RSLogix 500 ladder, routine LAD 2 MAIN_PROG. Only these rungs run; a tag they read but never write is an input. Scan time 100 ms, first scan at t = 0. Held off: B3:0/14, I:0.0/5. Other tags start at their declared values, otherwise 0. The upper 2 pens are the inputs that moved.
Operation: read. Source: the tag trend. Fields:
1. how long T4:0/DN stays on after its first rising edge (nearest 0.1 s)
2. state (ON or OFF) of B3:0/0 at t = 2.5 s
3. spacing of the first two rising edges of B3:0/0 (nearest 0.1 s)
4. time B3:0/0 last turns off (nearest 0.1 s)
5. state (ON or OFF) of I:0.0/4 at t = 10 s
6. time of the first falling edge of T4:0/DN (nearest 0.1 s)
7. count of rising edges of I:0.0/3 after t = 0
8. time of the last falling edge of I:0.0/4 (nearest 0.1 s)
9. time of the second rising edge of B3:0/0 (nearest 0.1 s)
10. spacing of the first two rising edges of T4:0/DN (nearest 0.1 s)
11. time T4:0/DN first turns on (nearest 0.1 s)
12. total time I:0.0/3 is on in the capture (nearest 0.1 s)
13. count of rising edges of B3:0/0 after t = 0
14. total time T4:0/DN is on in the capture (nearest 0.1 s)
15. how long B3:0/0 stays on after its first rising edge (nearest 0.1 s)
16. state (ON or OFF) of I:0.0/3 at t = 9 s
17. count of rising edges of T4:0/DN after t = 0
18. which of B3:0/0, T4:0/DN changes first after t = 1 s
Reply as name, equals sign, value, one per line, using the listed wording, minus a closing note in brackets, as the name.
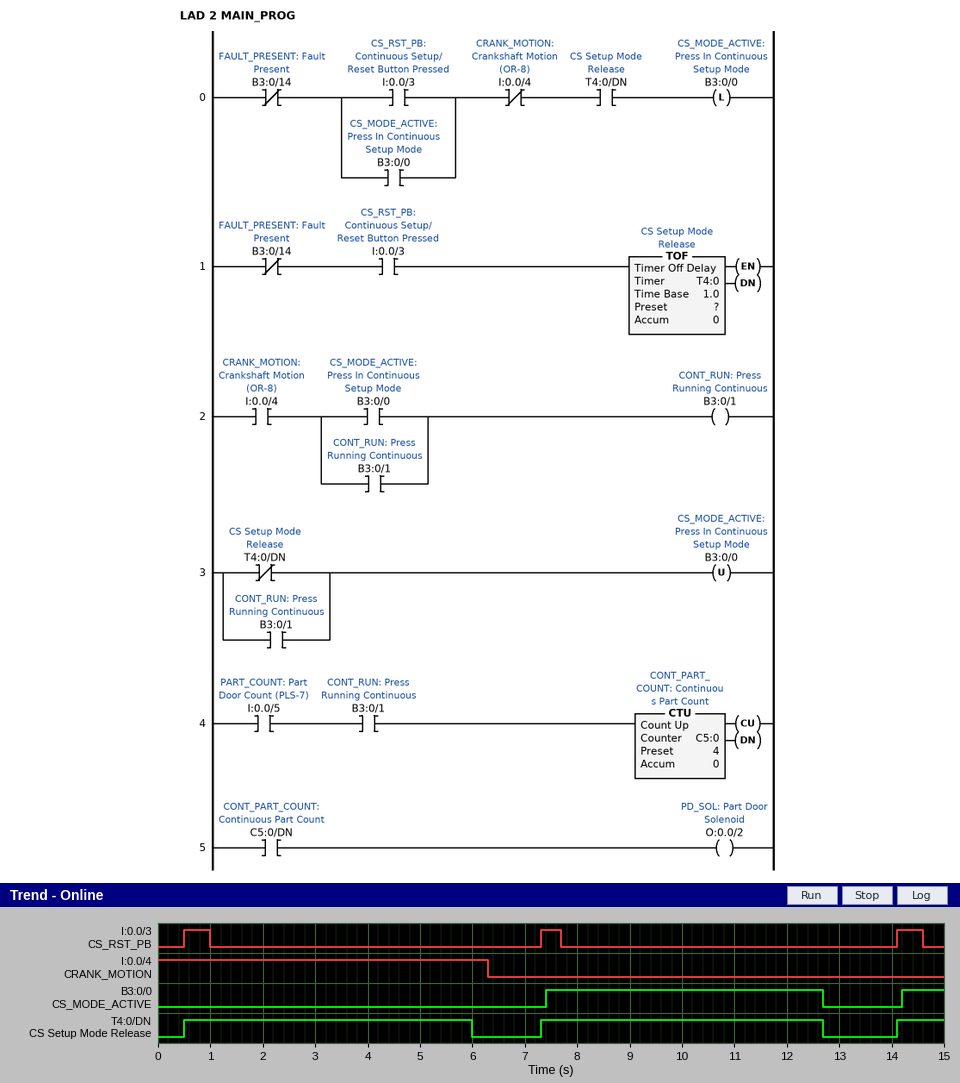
how long T4:0/DN stays on after its first rising edge = 5.5 s
state (ON or OFF) of B3:0/0 at t = 2.5 s = OFF
spacing of the first two rising edges of B3:0/0 = 6.8 s
time B3:0/0 last turns off = 12.7 s
state (ON or OFF) of I:0.0/4 at t = 10 s = OFF
time of the first falling edge of T4:0/DN = 6.0 s
count of rising edges of I:0.0/3 after t = 0 = 3
time of the last falling edge of I:0.0/4 = 6.3 s
time of the second rising edge of B3:0/0 = 14.2 s
spacing of the first two rising edges of T4:0/DN = 6.8 s
time T4:0/DN first turns on = 0.5 s
total time I:0.0/3 is on in the capture = 1.4 s
count of rising edges of B3:0/0 after t = 0 = 2
total time T4:0/DN is on in the capture = 11.8 s
how long B3:0/0 stays on after its first rising edge = 5.3 s
state (ON or OFF) of I:0.0/3 at t = 9 s = OFF
count of rising edges of T4:0/DN after t = 0 = 3
which of B3:0/0, T4:0/DN changes first after t = 1 s = T4:0/DN
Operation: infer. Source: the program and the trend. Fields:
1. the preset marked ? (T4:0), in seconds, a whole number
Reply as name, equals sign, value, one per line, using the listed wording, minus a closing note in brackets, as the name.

the preset marked ? (T4:0), in seconds, a whole number = 5 s
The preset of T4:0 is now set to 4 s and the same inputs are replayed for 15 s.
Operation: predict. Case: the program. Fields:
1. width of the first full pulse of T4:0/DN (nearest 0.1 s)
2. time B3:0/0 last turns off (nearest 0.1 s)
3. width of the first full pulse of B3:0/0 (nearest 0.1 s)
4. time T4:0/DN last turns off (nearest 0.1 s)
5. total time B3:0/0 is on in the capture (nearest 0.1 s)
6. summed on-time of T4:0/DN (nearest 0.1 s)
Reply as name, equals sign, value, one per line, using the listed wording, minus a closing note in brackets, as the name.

width of the first full pulse of T4:0/DN = 4.5 s
time B3:0/0 last turns off = 11.7 s
width of the first full pulse of B3:0/0 = 4.3 s
time T4:0/DN last turns off = 11.7 s
total time B3:0/0 is on in the capture = 5.1 s
summed on-time of T4:0/DN = 9.8 s
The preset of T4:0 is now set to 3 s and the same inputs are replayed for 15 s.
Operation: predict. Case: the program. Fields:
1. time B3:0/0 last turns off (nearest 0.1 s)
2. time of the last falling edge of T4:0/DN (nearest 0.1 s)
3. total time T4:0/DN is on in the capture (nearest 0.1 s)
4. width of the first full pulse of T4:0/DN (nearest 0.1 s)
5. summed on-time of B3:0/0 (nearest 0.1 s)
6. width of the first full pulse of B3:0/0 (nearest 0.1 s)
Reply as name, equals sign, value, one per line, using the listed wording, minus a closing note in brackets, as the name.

time B3:0/0 last turns off = 10.7 s
time of the last falling edge of T4:0/DN = 10.7 s
total time T4:0/DN is on in the capture = 7.8 s
width of the first full pulse of T4:0/DN = 3.5 s
summed on-time of B3:0/0 = 4.1 s
width of the first full pulse of B3:0/0 = 3.3 s
